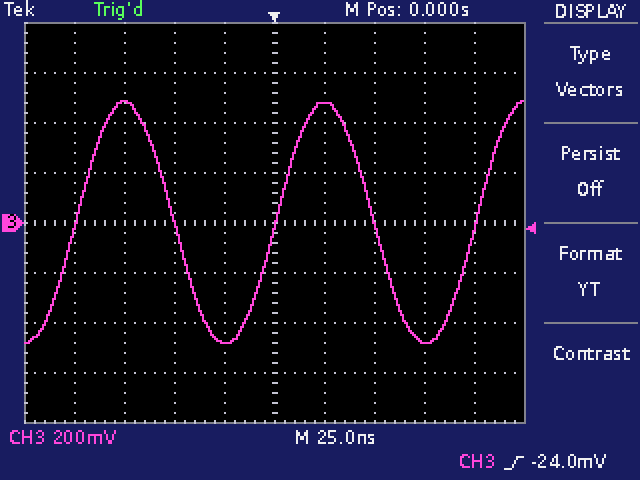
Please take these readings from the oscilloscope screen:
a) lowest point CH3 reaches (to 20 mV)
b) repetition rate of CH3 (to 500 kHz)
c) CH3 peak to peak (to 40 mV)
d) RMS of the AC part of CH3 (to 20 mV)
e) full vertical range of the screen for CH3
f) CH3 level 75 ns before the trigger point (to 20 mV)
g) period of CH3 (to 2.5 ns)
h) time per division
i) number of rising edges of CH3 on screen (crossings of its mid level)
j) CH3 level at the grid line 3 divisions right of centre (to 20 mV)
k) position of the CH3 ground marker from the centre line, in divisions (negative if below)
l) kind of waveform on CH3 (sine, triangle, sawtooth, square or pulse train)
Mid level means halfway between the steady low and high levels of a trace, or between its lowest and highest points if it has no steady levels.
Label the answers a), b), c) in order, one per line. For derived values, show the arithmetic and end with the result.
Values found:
a) -480 mV
b) 1 / 100.0 ns ≈ 10.0 MHz
c) 960 mV
d) 960 mV / (2√2) ≈ 339 mV, so 340 mV to the nearest 20 mV
e) 1.6 V
f) 480 mV
g) 100.0 ns
h) 25 ns
i) 3
j) -480 mV
k) 0.0 div
l) sine
